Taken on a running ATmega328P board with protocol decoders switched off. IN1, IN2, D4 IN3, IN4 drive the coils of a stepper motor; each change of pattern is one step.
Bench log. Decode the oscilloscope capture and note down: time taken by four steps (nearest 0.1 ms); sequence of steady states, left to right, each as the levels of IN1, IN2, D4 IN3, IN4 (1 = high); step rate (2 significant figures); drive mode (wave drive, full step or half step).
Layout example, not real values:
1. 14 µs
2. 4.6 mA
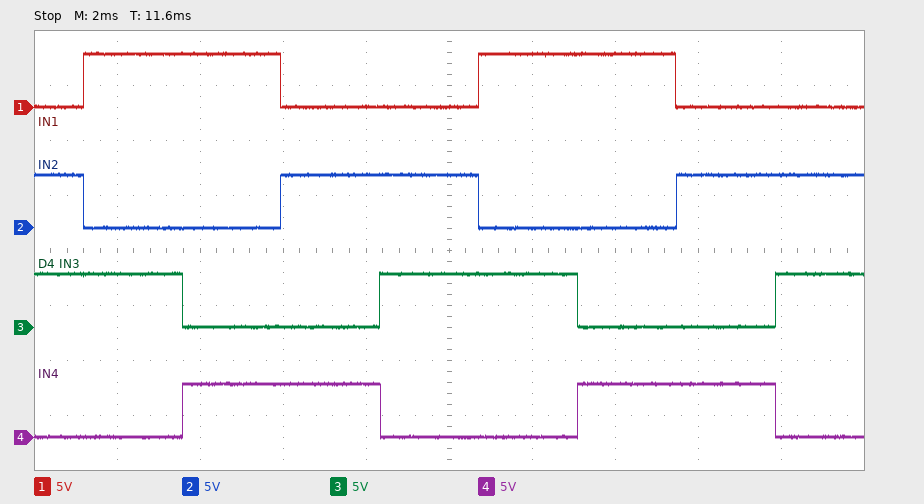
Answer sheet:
1. 9.5 ms
2. 0110 1010 1001 0101 0110 1010 1001 0101 0110
3. 420 steps/s
4. full step
